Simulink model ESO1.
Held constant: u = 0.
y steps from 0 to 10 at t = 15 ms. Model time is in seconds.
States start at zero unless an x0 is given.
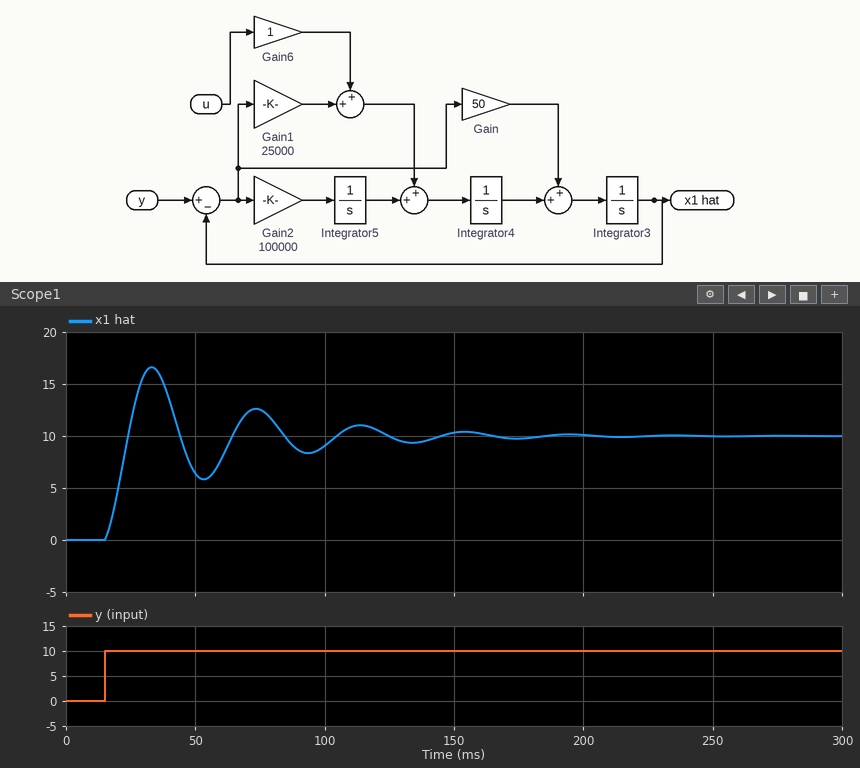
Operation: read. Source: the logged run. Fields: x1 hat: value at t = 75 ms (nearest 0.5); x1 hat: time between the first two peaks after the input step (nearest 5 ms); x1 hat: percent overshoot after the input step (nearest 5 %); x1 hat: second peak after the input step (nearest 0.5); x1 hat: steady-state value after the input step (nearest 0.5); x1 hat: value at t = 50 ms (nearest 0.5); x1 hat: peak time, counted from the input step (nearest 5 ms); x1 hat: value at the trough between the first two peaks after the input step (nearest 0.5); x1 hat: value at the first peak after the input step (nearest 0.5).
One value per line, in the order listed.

12.5
40 ms
65 %
12.5
10.0
6.5
20 ms
6.0
16.5
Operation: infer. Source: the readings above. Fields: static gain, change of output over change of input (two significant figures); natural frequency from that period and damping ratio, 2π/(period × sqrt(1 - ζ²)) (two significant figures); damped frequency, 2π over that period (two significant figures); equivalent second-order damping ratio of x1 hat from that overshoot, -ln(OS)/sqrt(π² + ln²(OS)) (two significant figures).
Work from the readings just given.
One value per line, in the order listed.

1.0
0.16 rad/ms
0.16 rad/ms
0.14
